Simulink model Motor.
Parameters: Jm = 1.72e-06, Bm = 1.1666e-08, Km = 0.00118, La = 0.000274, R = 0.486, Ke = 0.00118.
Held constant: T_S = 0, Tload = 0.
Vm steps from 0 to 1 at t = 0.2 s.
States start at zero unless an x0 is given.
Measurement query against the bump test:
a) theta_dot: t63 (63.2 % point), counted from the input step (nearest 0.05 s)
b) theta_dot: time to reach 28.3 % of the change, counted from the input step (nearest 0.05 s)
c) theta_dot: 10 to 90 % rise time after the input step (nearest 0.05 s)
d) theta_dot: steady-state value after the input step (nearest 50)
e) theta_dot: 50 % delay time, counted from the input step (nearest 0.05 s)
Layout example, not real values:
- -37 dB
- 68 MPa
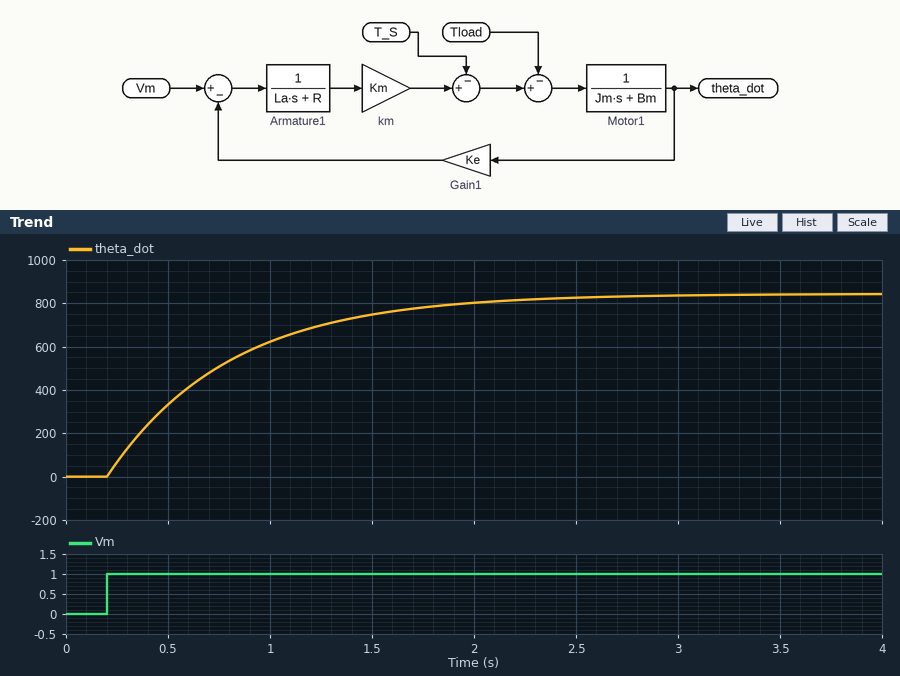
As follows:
- 0.60 s
- 0.20 s
- 1.30 s
- 850
- 0.40 s
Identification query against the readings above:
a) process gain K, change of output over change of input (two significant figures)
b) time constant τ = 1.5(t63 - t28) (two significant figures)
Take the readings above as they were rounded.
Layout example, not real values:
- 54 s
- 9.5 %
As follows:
- 850
- 0.60 s
